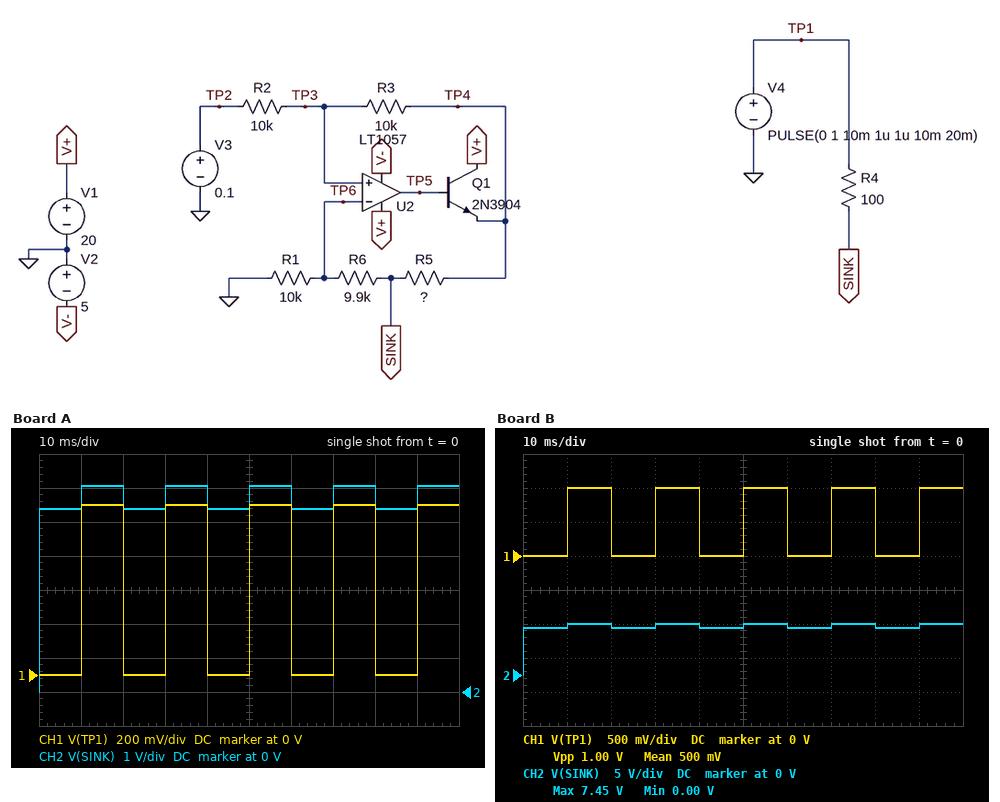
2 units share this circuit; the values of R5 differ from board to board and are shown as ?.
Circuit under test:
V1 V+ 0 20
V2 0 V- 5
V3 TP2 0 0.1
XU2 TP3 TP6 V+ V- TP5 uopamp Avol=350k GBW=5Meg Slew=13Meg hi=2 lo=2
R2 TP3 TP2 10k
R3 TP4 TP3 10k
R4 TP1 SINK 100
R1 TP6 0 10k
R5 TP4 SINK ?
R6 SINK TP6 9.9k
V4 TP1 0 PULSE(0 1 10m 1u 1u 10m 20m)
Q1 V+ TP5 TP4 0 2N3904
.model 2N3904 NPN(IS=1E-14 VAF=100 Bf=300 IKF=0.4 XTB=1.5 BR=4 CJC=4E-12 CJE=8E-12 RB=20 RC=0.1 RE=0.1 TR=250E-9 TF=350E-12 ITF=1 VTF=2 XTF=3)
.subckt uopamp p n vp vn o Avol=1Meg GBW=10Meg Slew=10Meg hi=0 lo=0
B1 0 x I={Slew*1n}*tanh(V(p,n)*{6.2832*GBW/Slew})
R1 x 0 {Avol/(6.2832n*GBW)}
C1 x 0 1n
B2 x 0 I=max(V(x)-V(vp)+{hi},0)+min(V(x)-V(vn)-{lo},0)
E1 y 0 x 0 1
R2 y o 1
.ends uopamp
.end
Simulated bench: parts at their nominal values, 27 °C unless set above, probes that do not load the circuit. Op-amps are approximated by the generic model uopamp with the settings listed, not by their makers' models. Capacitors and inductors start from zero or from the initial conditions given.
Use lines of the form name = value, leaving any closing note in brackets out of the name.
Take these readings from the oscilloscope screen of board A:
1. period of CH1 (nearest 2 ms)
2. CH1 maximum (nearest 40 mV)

period of CH1 = 20 ms
CH1 maximum = 1.00 V
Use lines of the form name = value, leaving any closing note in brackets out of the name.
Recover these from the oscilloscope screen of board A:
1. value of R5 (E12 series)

value of R5 = 220 Ω
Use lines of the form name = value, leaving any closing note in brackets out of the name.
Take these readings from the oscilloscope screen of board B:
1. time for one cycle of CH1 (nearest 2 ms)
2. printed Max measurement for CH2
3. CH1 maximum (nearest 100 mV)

time for one cycle of CH1 = 20 ms
printed Max measurement for CH2 = 7.45 V
CH1 maximum = 1.0 V
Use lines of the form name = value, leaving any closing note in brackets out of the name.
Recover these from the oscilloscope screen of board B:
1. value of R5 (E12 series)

value of R5 = 150 Ω
